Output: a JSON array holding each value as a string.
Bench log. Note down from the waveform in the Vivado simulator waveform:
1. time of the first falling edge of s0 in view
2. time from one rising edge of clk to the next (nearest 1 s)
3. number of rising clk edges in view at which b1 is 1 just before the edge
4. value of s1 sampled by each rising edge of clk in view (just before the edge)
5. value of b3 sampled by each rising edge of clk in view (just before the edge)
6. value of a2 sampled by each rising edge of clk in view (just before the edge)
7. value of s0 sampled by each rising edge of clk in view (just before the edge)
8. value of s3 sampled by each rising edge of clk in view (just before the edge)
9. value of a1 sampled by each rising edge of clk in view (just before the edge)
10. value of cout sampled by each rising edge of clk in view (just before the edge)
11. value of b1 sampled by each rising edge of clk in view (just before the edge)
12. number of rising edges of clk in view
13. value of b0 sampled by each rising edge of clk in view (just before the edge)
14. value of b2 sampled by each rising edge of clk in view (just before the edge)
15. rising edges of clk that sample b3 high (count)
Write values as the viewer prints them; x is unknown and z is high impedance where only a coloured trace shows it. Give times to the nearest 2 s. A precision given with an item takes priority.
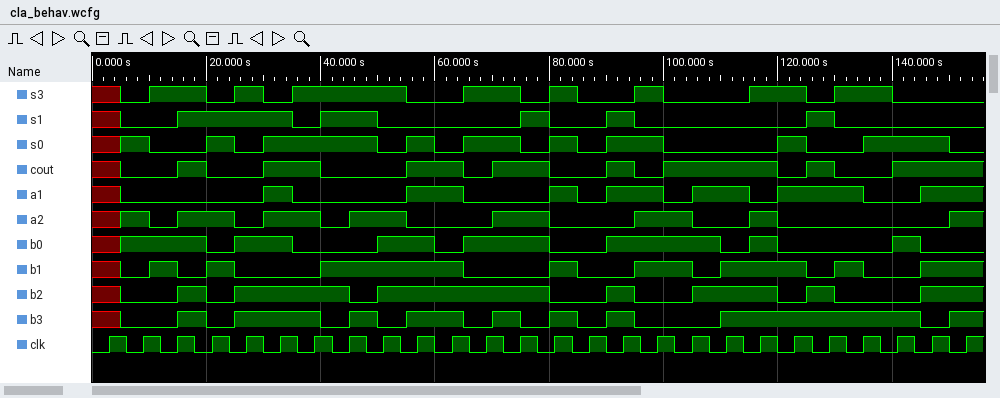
["10 s", "6 s", "15", "x 0 0 1 1 1 0 1 0 0 0 0 0 0 0 1 0 0 0 0 0 1 0 0 0 0", "x 0 0 0 1 1 1 0 0 1 1 0 1 1 0 1 0 0 1 1 1 1 1 1 0 1", "x 1 0 1 0 1 1 0 1 0 0 0 1 0 0 0 1 1 0 1 0 0 0 0 0 1", "x 1 0 1 0 1 1 1 0 1 0 1 1 1 0 1 1 0 0 0 1 0 0 1 1 0", "x 0 1 0 1 0 1 1 1 0 0 1 1 1 0 0 1 0 0 1 1 0 1 0 0 0", "x 0 0 0 0 1 0 0 0 1 1 0 0 1 0 1 1 0 1 0 1 1 1 0 1 1", "x 0 0 0 0 1 1 0 0 1 1 0 1 0 0 1 0 1 1 1 0 1 0 1 1 1", "x 0 1 1 0 0 0 1 1 1 1 0 0 1 0 0 1 1 1 1 1 0 1 0 1 1", "26", "x 1 1 0 1 1 0 0 1 1 0 1 1 0 0 1 1 1 0 1 0 0 0 1 0 0", "x 0 0 0 1 1 1 1 1 1 1 1 1 0 0 1 0 0 1 1 0 1 0 0 1 1", "15"]
